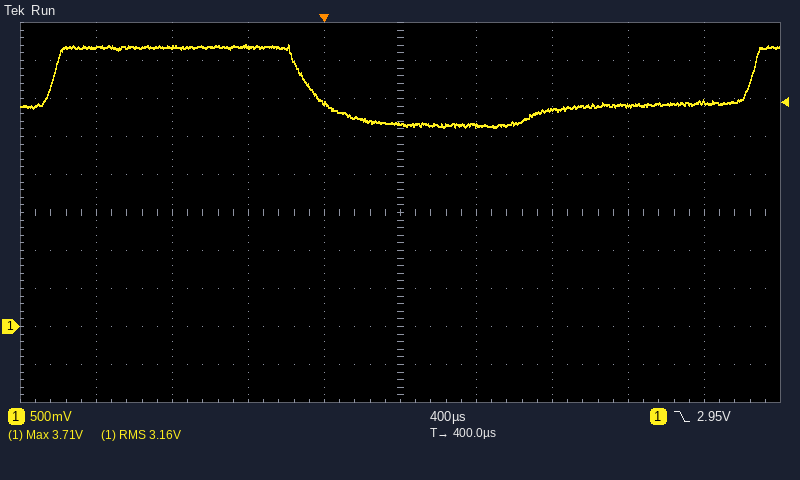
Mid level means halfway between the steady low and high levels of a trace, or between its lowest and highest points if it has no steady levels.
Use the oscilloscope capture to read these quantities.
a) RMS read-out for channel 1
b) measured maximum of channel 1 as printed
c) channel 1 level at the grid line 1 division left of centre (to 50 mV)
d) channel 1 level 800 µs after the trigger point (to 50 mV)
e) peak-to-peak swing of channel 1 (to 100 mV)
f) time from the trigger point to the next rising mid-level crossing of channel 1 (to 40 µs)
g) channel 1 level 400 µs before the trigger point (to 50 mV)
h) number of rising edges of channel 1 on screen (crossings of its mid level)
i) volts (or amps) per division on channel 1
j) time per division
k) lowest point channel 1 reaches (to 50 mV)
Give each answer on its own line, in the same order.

3.16 V
3.71 V
2.95 V
2.65 V
1.10 V
2.24 ms
3.70 V
2
500 mV
400 µs
2.60 V
